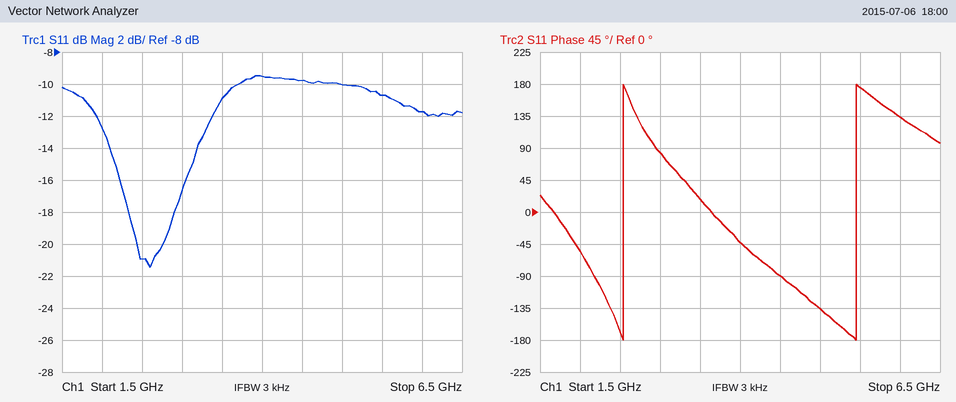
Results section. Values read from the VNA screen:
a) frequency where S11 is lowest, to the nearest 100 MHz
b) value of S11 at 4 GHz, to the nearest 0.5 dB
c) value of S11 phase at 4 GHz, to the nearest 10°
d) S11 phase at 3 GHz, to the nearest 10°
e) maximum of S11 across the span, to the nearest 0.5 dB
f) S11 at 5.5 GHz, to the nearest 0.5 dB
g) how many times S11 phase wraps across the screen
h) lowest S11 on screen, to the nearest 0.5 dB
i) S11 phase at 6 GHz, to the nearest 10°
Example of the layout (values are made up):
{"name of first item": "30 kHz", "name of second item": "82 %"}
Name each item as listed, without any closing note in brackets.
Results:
{"frequency where S11 is lowest, to the nearest 100 MHz": "2.6 GHz", "value of S11 at 4 GHz, to the nearest 0.5 dB": "-9.5 dB", "value of S11 phase at 4 GHz, to the nearest 10°": "-40°", "S11 phase at 3 GHz, to the nearest 10°": "80°", "maximum of S11 across the span, to the nearest 0.5 dB": "-9.5 dB", "S11 at 5.5 GHz, to the nearest 0.5 dB": "-10.5 dB", "how many times S11 phase wraps across the screen": "2", "lowest S11 on screen, to the nearest 0.5 dB": "-21.5 dB", "S11 phase at 6 GHz, to the nearest 10°": "130°"}
